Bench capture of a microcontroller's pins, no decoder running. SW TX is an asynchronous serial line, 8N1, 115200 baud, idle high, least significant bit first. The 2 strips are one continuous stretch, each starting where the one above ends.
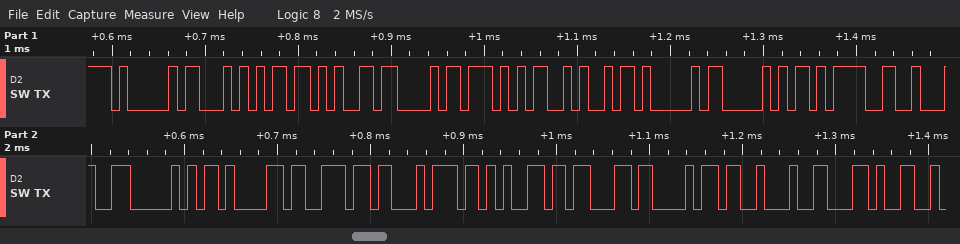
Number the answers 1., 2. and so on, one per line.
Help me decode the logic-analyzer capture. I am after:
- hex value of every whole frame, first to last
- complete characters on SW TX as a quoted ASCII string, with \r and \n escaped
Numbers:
1. 41 54 2B 43 57 4A 41 50 3D 22 50 61 6E 74 65 63 68 22 2C
2. "AT+CWJAP=\"Pantech\","
